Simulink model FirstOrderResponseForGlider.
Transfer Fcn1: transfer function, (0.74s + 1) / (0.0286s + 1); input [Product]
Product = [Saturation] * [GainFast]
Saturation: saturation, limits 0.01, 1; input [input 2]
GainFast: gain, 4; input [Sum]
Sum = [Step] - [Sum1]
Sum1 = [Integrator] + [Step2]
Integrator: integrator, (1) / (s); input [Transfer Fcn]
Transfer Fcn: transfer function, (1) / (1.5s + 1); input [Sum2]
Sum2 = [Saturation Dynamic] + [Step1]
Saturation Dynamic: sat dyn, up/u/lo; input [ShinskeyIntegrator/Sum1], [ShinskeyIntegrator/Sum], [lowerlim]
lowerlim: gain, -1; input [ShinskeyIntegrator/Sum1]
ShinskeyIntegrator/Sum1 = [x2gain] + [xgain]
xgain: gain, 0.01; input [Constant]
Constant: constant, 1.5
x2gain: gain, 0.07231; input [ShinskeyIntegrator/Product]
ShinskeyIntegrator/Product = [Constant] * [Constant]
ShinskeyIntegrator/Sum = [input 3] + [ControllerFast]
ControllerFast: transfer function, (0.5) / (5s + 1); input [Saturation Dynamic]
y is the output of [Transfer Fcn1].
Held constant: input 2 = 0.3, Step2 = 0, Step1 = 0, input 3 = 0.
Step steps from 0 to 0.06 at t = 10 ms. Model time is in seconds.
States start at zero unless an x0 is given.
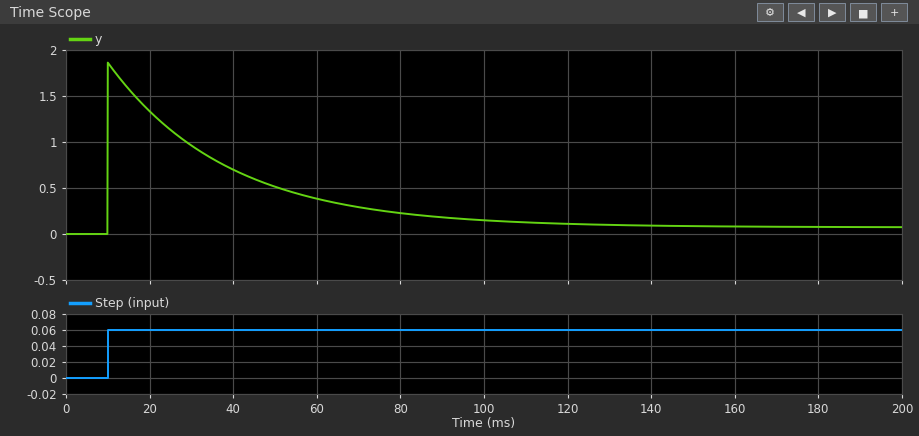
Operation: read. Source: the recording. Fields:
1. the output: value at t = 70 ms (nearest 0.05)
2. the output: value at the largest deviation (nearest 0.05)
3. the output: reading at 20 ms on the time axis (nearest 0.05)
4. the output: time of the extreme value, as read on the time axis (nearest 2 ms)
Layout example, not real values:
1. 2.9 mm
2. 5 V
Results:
1. 0.30
2. 1.85
3. 1.35
4. 10 ms
